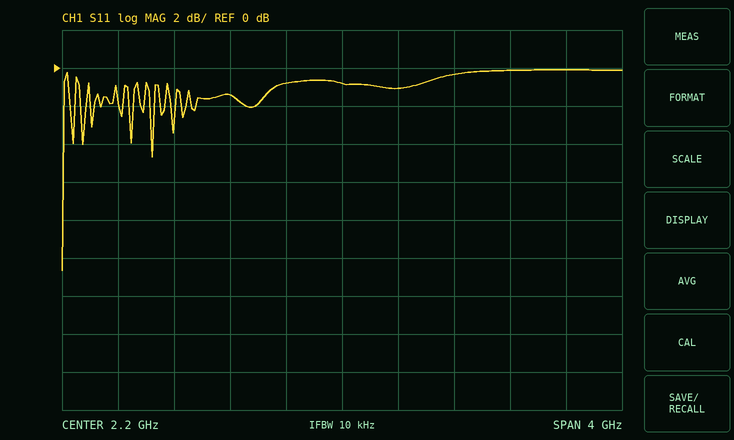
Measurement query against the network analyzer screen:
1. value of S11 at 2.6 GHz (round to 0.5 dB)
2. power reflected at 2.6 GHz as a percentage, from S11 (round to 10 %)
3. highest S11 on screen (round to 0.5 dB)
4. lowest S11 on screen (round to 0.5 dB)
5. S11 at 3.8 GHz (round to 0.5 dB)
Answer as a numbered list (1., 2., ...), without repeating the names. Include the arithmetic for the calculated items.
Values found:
1. -1.0 dB
2. 10^(-1/10) ≈ 79.4 %, so 80 % to the nearest 10 %
3. 0.0 dB
4. -10.5 dB
5. 0.0 dB
